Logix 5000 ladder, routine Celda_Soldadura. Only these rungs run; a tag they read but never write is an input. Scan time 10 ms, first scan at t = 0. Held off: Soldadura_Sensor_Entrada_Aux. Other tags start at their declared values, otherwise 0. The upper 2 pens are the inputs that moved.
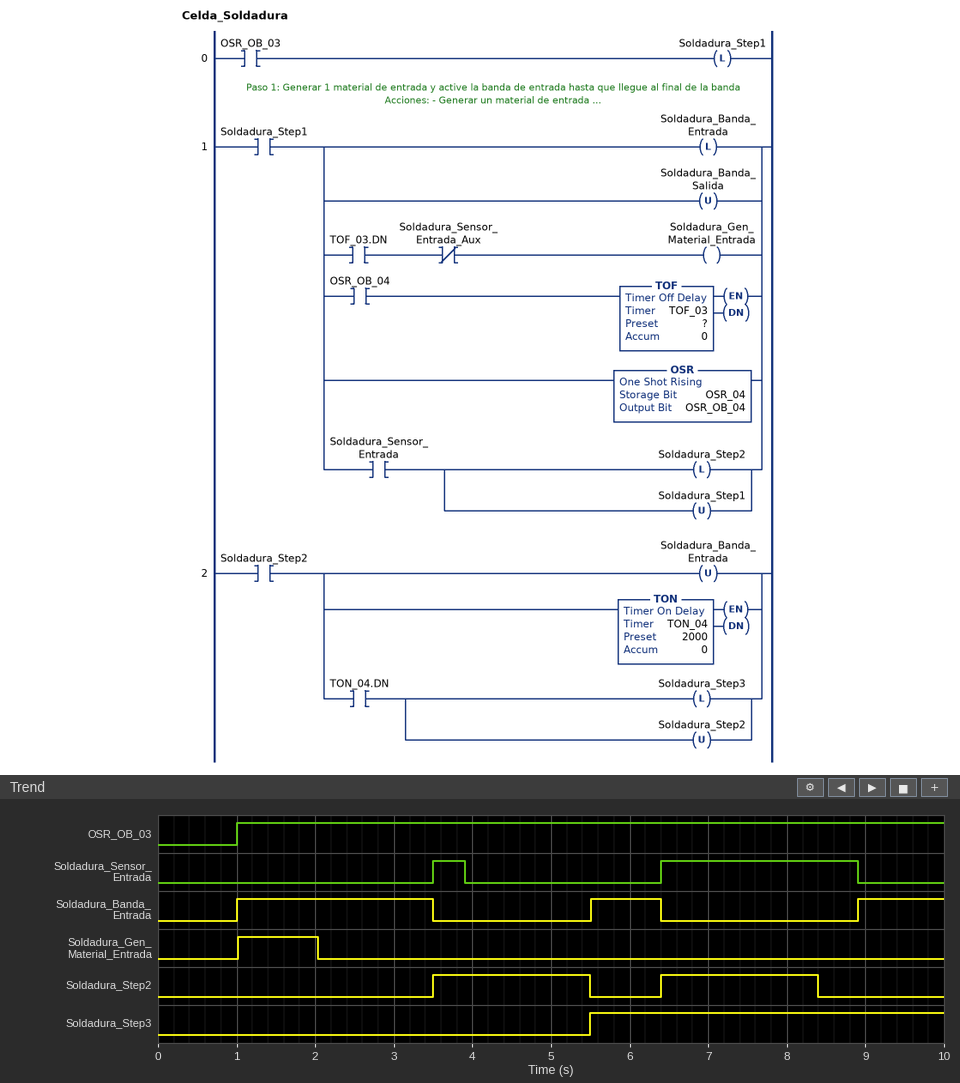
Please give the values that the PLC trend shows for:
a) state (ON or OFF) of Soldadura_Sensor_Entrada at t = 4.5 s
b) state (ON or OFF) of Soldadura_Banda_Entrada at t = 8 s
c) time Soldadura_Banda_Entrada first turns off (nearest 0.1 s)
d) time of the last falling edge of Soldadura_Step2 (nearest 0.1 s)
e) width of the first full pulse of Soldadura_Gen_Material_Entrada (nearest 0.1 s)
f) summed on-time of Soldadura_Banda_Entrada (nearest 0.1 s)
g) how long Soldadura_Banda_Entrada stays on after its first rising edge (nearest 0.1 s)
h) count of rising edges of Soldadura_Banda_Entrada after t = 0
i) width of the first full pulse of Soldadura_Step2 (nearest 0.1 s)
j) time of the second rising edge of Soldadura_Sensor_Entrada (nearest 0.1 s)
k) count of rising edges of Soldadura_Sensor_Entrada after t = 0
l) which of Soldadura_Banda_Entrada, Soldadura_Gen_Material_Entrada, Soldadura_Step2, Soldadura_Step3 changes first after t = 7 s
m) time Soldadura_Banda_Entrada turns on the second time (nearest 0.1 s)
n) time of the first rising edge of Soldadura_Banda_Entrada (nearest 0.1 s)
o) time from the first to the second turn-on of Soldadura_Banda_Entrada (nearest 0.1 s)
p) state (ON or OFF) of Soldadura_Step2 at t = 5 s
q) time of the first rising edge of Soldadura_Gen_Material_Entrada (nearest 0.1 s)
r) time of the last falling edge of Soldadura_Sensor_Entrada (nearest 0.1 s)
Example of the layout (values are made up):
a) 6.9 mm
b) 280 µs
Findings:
a) OFF
b) OFF
c) 3.5 s
d) 8.4 s
e) 1.0 s
f) 4.5 s
g) 2.5 s
h) 3
i) 2.0 s
j) 6.4 s
k) 2
l) Soldadura_Step2
m) 5.5 s
n) 1.0 s
o) 4.5 s
p) ON
q) 1.0 s
r) 8.9 s
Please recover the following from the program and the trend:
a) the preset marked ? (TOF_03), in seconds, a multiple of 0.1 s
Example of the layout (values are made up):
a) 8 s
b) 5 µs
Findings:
a) 1.0 s
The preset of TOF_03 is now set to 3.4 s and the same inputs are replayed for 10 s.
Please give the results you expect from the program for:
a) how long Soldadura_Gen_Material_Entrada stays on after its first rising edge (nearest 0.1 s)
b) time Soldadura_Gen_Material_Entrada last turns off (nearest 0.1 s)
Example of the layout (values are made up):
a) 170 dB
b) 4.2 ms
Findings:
a) 3.4 s
b) 4.4 s
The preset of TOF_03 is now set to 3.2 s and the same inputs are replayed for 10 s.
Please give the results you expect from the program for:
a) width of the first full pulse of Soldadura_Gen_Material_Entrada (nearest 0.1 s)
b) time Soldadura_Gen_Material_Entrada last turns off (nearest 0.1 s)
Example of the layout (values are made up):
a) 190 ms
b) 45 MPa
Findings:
a) 3.2 s
b) 4.2 s
